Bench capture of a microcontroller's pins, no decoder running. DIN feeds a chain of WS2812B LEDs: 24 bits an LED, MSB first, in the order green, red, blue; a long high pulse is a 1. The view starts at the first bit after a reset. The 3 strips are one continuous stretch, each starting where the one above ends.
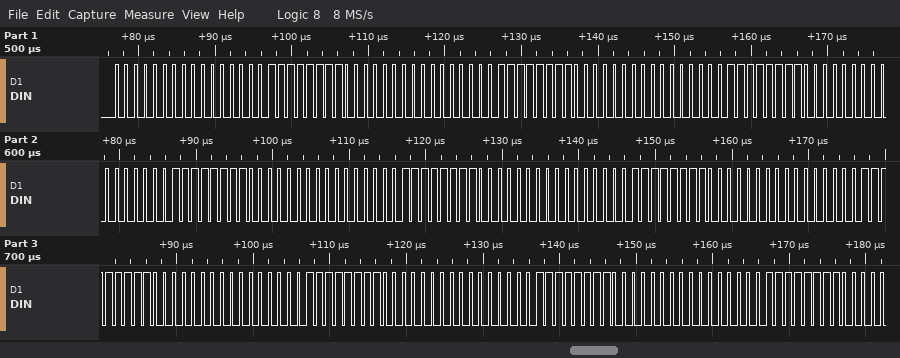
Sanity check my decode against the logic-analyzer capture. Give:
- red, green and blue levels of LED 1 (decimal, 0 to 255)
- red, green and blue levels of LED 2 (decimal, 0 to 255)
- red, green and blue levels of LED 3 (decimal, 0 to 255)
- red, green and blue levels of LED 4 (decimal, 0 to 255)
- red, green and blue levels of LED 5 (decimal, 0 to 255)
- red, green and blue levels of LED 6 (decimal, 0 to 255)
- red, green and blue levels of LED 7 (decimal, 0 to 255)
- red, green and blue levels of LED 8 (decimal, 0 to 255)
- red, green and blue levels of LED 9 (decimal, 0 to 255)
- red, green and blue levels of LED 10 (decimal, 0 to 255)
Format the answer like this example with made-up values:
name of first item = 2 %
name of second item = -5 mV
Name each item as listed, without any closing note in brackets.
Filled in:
red, green and blue levels of LED 1 = 0, 0, 255
red, green and blue levels of LED 2 = 0, 0, 255
red, green and blue levels of LED 3 = 0, 0, 255
red, green and blue levels of LED 4 = 0, 0, 255
red, green and blue levels of LED 5 = 0, 0, 255
red, green and blue levels of LED 6 = 0, 0, 255
red, green and blue levels of LED 7 = 0, 0, 255
red, green and blue levels of LED 8 = 0, 0, 255
red, green and blue levels of LED 9 = 0, 0, 255
red, green and blue levels of LED 10 = 0, 0, 255
